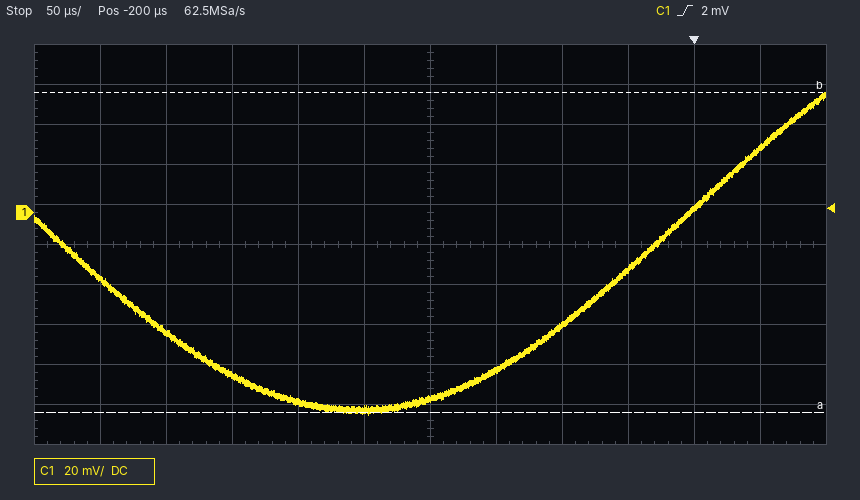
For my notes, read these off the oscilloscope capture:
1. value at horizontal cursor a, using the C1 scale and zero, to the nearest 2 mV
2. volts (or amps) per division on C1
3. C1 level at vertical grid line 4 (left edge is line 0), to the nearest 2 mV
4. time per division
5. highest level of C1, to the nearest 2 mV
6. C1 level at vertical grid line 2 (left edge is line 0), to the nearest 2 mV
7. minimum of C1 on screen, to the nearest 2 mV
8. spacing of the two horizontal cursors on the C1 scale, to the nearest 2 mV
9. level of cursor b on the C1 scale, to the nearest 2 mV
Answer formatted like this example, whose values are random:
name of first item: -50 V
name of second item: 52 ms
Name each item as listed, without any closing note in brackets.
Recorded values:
value at horizontal cursor a, using the C1 scale and zero, to the nearest 2 mV: -100 mV
volts (or amps) per division on C1: 20 mV
C1 level at vertical grid line 4 (left edge is line 0), to the nearest 2 mV: -94 mV
time per division: 50 µs
highest level of C1, to the nearest 2 mV: 60 mV
C1 level at vertical grid line 2 (left edge is line 0), to the nearest 2 mV: -60 mV
minimum of C1 on screen, to the nearest 2 mV: -100 mV
spacing of the two horizontal cursors on the C1 scale, to the nearest 2 mV: 160 mV
level of cursor b on the C1 scale, to the nearest 2 mV: 60 mV
